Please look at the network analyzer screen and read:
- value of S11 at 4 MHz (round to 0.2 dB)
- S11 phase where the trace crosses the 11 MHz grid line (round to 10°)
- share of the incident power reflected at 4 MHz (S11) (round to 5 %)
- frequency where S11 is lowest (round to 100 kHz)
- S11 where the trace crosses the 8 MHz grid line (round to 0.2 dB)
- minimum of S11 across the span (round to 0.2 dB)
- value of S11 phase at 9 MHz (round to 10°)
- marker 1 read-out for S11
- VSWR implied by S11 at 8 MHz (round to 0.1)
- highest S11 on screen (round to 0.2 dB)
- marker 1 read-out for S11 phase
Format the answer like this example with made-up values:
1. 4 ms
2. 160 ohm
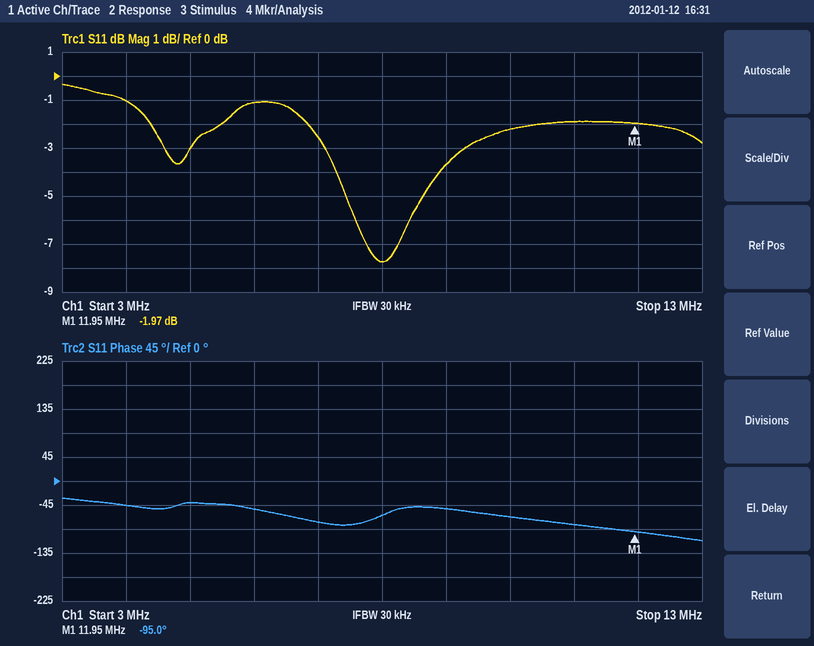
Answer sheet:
1. -1.0 dB
2. -80°
3. 80 %
4. 8.0 MHz
5. -7.8 dB
6. -7.8 dB
7. -50°
8. -1.97 dB
9. 2.4
10. -0.4 dB
11. -95.0°
